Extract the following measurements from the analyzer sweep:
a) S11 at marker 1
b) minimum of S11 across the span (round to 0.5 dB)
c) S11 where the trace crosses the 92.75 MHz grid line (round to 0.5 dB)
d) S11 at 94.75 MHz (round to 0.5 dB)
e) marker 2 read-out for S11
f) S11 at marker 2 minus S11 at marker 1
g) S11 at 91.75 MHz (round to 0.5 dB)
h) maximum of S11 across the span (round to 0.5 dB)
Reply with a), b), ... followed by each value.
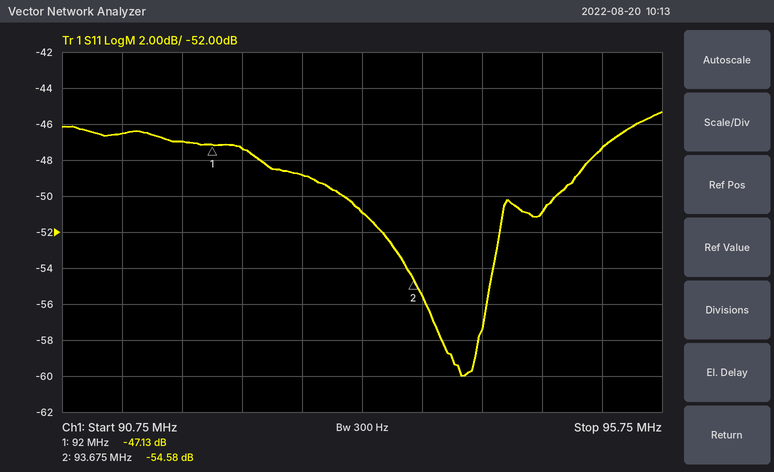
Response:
a) -47.13 dB
b) -60.0 dB
c) -49.0 dB
d) -51.0 dB
e) -54.58 dB
f) -7.45 dB
g) -47.0 dB
h) -45.5 dB
